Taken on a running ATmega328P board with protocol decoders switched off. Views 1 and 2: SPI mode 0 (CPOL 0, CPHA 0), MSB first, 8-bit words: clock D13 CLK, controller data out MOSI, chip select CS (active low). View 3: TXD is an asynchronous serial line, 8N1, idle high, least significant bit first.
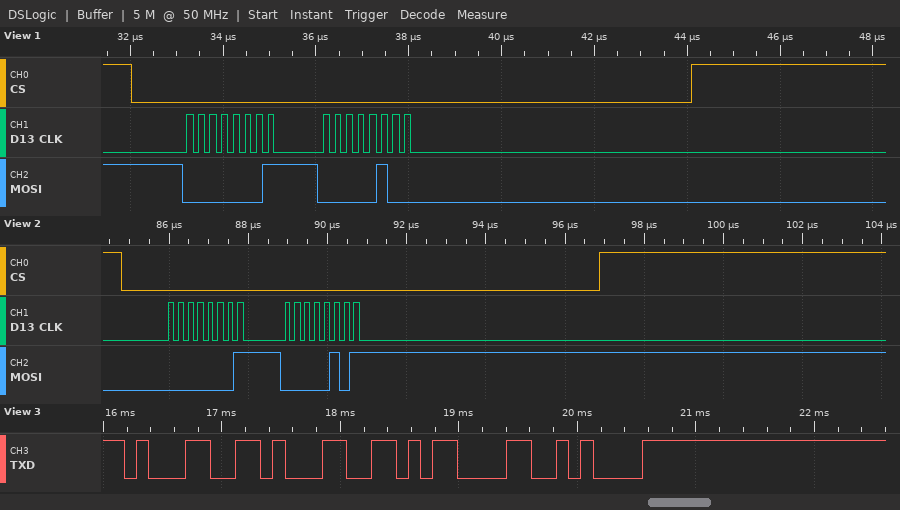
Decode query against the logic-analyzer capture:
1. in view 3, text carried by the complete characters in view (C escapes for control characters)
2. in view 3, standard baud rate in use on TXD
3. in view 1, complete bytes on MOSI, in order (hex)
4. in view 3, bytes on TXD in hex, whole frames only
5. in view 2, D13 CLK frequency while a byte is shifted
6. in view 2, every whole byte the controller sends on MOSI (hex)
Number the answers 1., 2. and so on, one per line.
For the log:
1. "11\r\n"
2. 9600 baud
3. 01 04
4. 0x31 0x31 0x0D 0x0A
5. 4 MHz
6. 0x01 0x05
